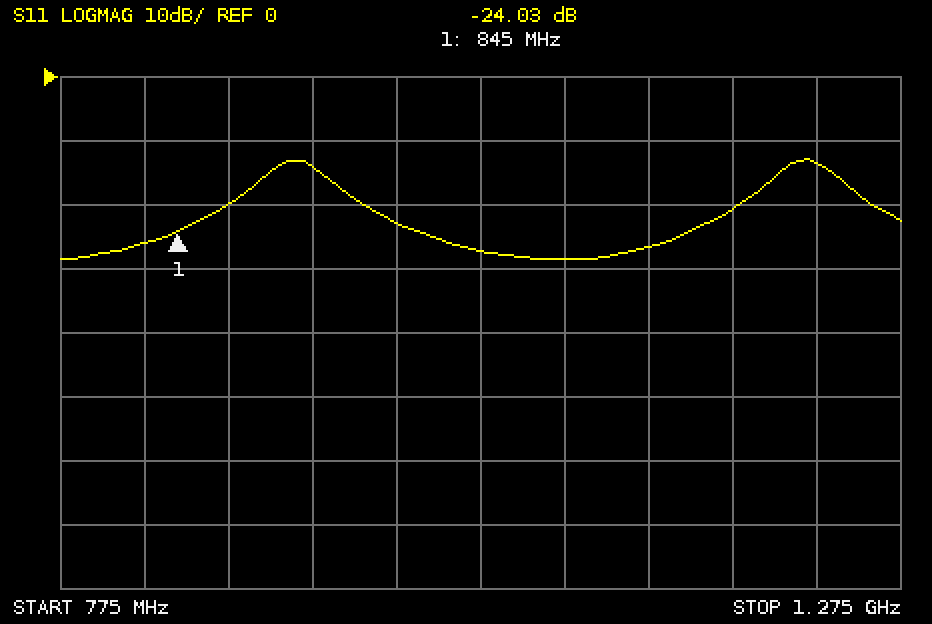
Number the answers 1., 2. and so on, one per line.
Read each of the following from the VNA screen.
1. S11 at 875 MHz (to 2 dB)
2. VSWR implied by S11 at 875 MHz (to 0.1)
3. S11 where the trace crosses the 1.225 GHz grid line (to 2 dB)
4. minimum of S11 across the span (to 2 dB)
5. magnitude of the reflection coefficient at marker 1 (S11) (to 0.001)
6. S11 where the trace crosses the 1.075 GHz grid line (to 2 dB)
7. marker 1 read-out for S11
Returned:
1. -20 dB
2. 1.2
3. -14 dB
4. -28 dB
5. 0.063
6. -28 dB
7. -24.03 dB
